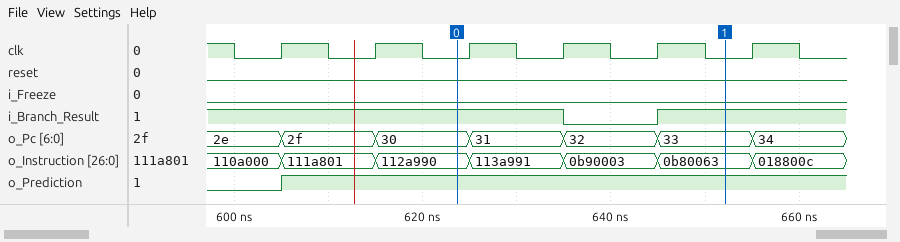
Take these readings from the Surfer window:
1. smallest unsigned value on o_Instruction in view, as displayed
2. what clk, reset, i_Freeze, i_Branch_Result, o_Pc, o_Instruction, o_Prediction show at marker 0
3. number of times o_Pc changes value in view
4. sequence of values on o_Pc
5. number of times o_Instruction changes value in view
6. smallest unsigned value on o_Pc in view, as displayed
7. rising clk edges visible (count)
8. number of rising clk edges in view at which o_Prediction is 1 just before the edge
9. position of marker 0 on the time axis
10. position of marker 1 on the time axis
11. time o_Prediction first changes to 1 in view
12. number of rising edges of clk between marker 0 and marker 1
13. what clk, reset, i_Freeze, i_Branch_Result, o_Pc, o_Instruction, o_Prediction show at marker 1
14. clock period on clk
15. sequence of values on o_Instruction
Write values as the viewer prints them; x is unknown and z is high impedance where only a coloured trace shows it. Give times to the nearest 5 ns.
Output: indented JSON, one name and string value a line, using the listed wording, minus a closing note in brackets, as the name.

{
  "smallest unsigned value on o_Instruction in view, as displayed": "018800c",
  "what clk, reset, i_Freeze, i_Branch_Result, o_Pc, o_Instruction, o_Prediction show at marker 0": "clk=0, reset=0, i_Freeze=0, i_Branch_Result=1, o_Pc=30, o_Instruction=112a990, o_Prediction=1",
  "number of times o_Pc changes value in view": "6",
  "sequence of values on o_Pc": "2e, 2f, 30, 31, 32, 33, 34",
  "number of times o_Instruction changes value in view": "6",
  "smallest unsigned value on o_Pc in view, as displayed": "2e",
  "rising clk edges visible": "6",
  "number of rising clk edges in view at which o_Prediction is 1 just before the edge": "5",
  "position of marker 0 on the time axis": "625 ns",
  "position of marker 1 on the time axis": "650 ns",
  "time o_Prediction first changes to 1 in view": "605 ns",
  "number of rising edges of clk between marker 0 and marker 1": "3",
  "what clk, reset, i_Freeze, i_Branch_Result, o_Pc, o_Instruction, o_Prediction show at marker 1": "clk=0, reset=0, i_Freeze=0, i_Branch_Result=1, o_Pc=33, o_Instruction=0b80063, o_Prediction=1",
  "clock period on clk": "10 ns",
  "sequence of values on o_Instruction": "110a000, 111a801, 112a990, 113a991, 0b90003, 0b80063, 018800c"
}
